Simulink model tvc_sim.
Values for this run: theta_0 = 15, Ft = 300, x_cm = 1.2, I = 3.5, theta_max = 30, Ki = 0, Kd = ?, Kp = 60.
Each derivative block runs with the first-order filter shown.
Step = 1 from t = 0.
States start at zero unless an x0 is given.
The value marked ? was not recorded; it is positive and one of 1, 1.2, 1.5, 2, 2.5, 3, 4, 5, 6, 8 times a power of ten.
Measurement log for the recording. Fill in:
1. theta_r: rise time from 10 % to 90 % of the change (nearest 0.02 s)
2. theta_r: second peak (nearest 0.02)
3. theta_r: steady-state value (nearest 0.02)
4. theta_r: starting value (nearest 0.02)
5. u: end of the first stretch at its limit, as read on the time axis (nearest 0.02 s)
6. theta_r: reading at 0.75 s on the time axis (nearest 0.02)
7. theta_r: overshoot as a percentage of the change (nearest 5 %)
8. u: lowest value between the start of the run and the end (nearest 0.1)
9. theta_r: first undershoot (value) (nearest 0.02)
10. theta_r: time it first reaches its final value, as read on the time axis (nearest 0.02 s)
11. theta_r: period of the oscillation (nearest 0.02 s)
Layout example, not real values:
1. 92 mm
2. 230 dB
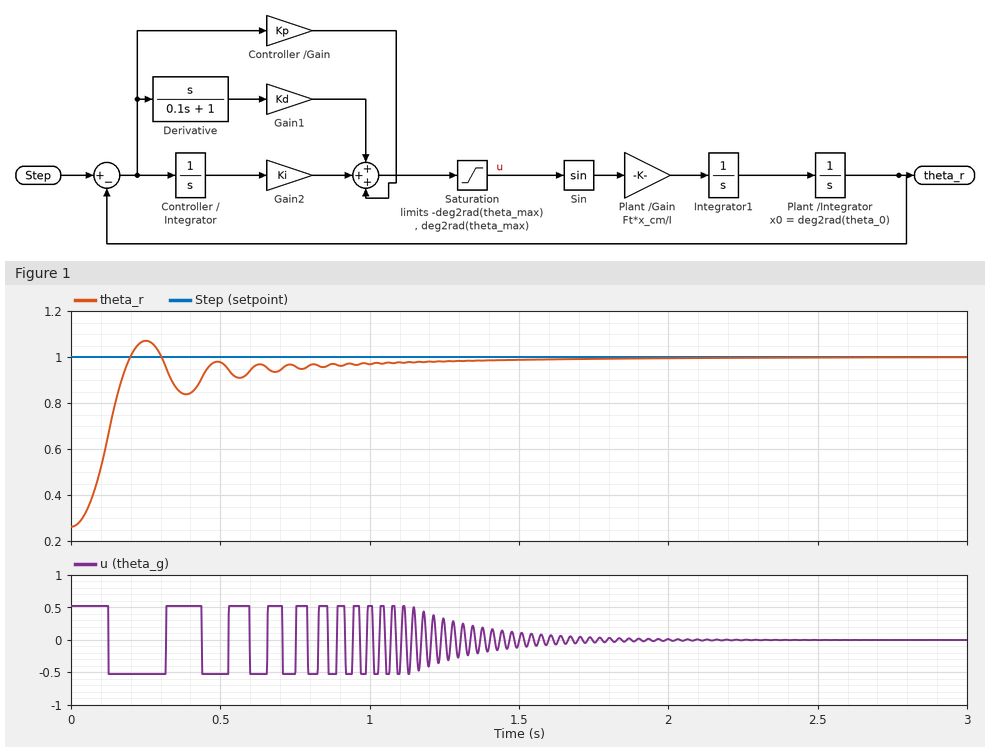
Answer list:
1. 0.12 s
2. 0.98
3. 1.00
4. 0.26
5. 0.12 s
6. 0.96
7. 10 %
8. -0.5
9. 0.84
10. 0.20 s
11. 0.24 s
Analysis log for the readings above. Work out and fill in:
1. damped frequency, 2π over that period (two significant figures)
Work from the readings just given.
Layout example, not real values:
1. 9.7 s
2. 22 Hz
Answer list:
1. 26 rad/s
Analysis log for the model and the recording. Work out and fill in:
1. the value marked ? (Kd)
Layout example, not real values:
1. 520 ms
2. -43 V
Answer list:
1. 30
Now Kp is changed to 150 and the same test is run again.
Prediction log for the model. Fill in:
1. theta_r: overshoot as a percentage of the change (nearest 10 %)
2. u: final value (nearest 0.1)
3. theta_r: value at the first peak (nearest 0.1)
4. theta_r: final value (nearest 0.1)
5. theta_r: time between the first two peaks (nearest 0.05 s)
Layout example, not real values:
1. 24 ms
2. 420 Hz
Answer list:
1. 30 %
2. 0.0
3. 1.2
4. 1.0
5. 0.30 s
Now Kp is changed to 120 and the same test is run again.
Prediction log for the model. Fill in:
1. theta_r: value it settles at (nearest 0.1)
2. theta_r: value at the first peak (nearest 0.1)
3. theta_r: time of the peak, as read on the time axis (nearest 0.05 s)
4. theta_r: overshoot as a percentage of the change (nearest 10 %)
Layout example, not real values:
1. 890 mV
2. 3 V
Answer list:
1. 1.0
2. 1.2
3. 0.25 s
4. 20 %
